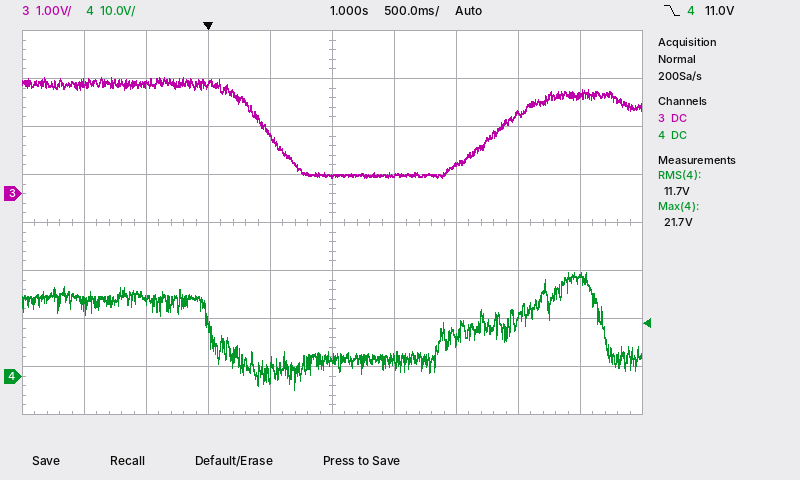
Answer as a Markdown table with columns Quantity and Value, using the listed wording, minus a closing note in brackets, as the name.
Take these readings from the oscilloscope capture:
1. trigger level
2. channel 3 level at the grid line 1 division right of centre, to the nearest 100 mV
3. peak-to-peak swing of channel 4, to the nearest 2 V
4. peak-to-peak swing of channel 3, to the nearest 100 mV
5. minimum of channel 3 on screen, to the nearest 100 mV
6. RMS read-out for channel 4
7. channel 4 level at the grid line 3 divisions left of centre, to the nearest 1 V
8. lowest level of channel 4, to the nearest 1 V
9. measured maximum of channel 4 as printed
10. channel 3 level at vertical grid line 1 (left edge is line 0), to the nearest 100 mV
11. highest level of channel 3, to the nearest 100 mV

| Quantity | Value |
|---|---|
| trigger level | 11.0 V |
| channel 3 level at the grid line 1 division right of centre, to the nearest 100 mV | 400 mV |
| peak-to-peak swing of channel 4, to the nearest 2 V | 24 V |
| peak-to-peak swing of channel 3, to the nearest 100 mV | 2.1 V |
| minimum of channel 3 on screen, to the nearest 100 mV | 300 mV |
| RMS read-out for channel 4 | 11.7 V |
| channel 4 level at the grid line 3 divisions left of centre, to the nearest 1 V | 16 V |
| lowest level of channel 4, to the nearest 1 V | -3 V |
| measured maximum of channel 4 as printed | 21.7 V |
| channel 3 level at vertical grid line 1 (left edge is line 0), to the nearest 100 mV | 2.3 V |
| highest level of channel 3, to the nearest 100 mV | 2.4 V |
